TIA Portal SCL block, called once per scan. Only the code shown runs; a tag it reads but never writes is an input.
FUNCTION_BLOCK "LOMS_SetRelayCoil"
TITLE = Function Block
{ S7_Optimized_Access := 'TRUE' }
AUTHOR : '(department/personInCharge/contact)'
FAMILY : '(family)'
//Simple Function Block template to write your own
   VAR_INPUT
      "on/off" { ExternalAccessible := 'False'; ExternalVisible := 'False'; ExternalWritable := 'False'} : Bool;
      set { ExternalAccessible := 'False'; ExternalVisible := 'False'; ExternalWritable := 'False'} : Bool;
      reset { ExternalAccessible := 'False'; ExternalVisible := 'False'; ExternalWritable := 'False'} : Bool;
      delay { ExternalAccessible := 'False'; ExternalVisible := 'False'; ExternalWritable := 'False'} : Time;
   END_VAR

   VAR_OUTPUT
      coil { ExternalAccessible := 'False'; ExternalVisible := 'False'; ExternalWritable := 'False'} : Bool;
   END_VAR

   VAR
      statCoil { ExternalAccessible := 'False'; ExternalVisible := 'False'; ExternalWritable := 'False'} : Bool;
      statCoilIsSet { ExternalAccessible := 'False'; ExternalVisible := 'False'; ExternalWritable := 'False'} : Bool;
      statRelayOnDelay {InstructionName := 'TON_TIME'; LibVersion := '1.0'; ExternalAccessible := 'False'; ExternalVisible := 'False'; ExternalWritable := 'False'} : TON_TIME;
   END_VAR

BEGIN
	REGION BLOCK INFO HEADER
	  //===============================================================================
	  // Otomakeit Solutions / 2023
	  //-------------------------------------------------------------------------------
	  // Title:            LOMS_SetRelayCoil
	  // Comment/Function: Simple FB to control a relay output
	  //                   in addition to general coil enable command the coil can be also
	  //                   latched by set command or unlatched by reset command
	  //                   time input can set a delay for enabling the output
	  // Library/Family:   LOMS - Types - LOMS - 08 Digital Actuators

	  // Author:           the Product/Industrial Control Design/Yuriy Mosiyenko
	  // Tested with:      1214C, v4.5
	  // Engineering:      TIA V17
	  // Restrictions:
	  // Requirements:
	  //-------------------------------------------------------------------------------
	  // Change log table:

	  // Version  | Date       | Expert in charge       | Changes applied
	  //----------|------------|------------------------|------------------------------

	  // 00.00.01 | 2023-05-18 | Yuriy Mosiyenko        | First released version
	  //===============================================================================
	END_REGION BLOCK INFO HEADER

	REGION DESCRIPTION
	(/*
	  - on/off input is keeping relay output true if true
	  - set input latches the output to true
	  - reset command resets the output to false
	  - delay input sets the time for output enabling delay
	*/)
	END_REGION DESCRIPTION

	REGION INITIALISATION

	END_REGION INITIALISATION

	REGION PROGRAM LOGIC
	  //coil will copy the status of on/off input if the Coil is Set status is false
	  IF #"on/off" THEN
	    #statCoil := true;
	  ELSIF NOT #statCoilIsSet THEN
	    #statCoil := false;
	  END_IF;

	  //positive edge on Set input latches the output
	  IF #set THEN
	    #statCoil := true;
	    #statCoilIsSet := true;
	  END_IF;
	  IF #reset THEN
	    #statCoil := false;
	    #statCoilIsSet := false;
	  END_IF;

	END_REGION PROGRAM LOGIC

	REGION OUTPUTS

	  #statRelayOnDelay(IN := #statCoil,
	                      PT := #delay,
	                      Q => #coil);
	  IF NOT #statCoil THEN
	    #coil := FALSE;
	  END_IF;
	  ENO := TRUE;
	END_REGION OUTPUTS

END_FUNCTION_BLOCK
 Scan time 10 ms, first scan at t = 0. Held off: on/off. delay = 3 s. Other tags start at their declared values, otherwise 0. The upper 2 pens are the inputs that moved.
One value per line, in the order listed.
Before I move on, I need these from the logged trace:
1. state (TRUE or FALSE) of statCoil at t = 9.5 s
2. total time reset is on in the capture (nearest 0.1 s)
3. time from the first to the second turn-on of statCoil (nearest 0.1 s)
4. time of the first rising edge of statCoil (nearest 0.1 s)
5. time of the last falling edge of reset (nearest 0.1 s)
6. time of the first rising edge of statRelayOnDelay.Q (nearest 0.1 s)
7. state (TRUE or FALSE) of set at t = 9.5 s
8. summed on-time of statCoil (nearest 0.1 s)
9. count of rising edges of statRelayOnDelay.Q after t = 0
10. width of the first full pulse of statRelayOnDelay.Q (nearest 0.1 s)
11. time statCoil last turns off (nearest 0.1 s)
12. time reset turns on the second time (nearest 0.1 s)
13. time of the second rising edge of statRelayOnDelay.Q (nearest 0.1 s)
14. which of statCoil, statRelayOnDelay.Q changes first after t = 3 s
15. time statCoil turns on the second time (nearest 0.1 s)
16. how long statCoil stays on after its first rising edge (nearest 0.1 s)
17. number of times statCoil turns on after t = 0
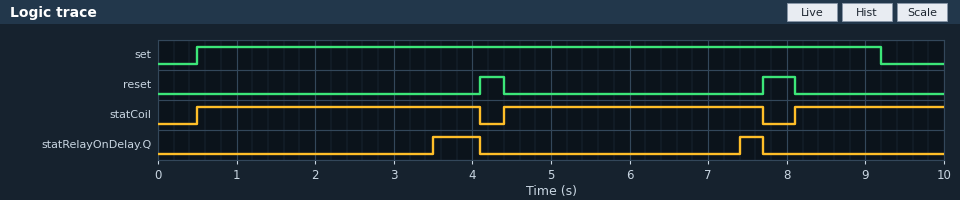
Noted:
TRUE
0.7 s
3.9 s
0.5 s
8.1 s
3.5 s
FALSE
8.8 s
2
0.6 s
7.7 s
7.7 s
7.4 s
statRelayOnDelay.Q
4.4 s
3.6 s
3
